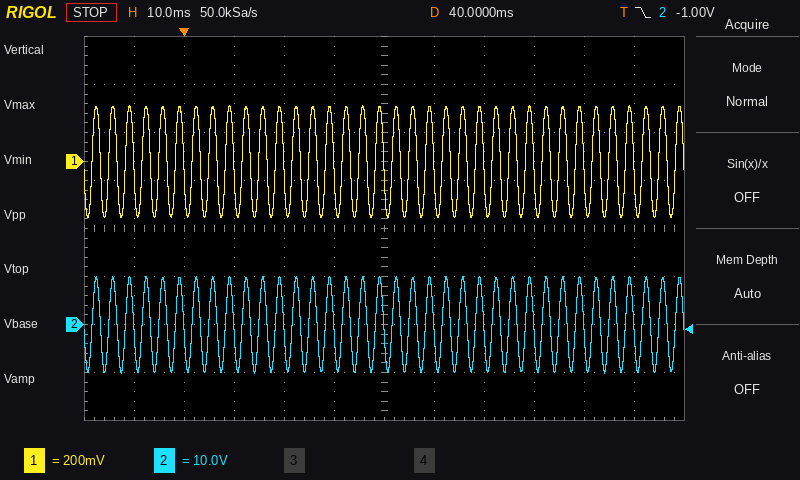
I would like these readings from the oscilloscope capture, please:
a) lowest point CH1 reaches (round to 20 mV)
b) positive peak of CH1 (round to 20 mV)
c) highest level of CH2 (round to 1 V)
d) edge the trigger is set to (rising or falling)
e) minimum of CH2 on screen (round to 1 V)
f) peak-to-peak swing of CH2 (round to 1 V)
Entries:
-240 mV
240 mV
10 V
falling
-10 V
20 V
